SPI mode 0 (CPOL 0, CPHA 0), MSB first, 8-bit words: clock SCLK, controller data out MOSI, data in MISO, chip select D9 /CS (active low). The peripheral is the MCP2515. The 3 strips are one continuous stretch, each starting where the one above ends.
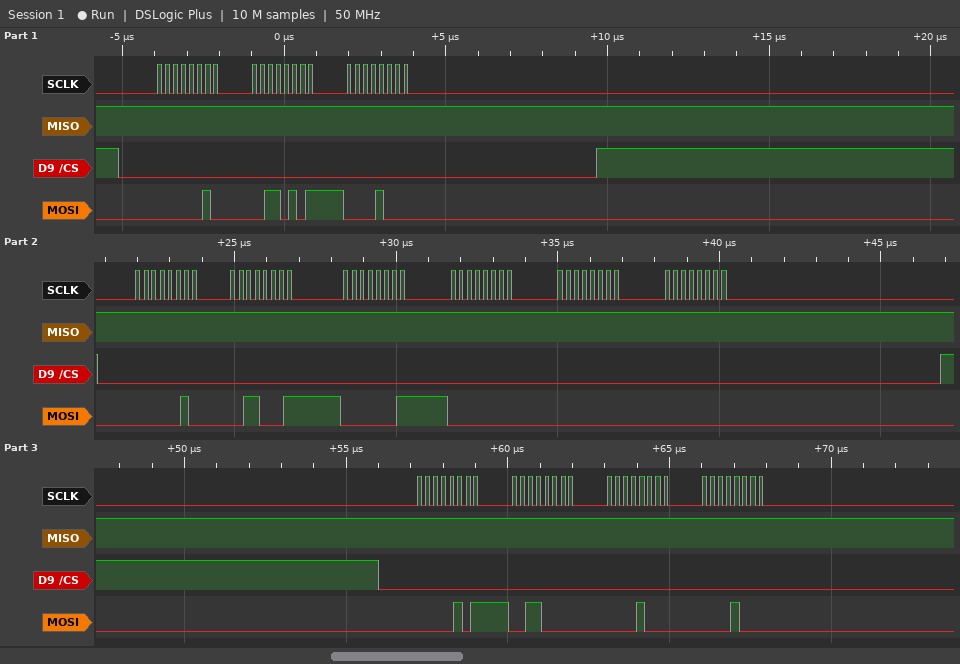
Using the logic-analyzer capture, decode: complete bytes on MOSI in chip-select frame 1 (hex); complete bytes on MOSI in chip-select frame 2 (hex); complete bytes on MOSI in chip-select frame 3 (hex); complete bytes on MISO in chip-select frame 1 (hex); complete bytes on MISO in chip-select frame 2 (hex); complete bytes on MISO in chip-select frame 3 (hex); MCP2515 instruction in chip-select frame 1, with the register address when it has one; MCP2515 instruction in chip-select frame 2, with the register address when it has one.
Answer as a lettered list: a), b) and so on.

a) 0x02 0x35 0x08
b) 0x02 0x31 0x01 0x00 0x00 0x00
c) 0x05 0x30 0x08 0x08
d) 0xFF 0xFF 0xFF
e) 0xFF 0xFF 0xFF 0xFF 0xFF 0xFF
f) 0xFF 0xFF 0xFF 0xFF
g) WRITE 0x35
h) WRITE 0x31
